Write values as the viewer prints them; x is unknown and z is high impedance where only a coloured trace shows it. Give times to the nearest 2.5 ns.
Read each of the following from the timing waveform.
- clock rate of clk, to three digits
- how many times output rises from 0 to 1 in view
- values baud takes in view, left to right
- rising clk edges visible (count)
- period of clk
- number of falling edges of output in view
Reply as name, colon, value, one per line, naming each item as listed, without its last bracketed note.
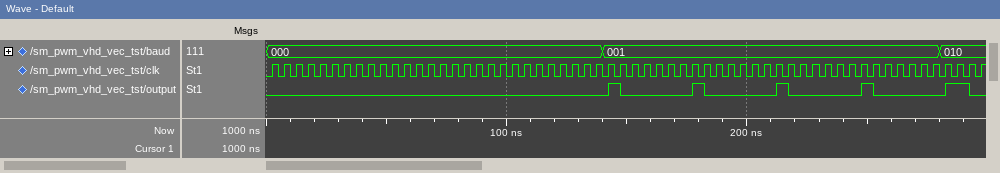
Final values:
clock rate of clk, to three digits: 200 MHz
how many times output rises from 0 to 1 in view: 5
values baud takes in view, left to right: 000, 001, 010
rising clk edges visible: 60
period of clk: 5 ns
number of falling edges of output in view: 5
